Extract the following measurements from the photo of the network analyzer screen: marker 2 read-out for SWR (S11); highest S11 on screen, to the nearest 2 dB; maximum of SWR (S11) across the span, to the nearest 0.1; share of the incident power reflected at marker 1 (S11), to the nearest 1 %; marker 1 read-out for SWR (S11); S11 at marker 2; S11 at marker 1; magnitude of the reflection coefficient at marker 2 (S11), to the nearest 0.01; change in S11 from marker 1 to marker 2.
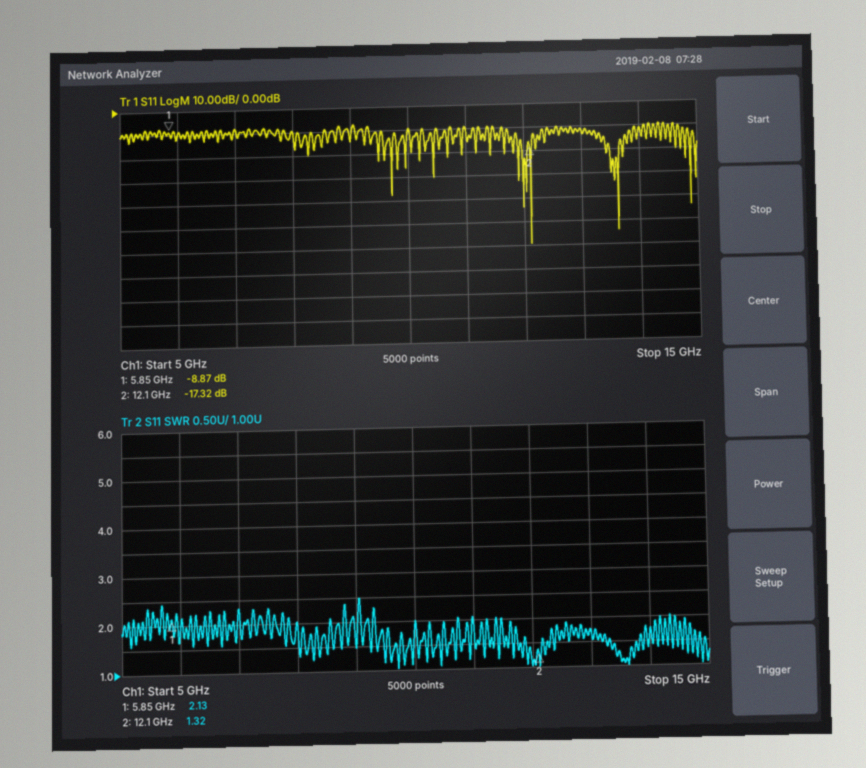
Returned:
1.32
-8 dB
2.5
13 %
2.13
-17.32 dB
-8.87 dB
0.14
-8.45 dB
